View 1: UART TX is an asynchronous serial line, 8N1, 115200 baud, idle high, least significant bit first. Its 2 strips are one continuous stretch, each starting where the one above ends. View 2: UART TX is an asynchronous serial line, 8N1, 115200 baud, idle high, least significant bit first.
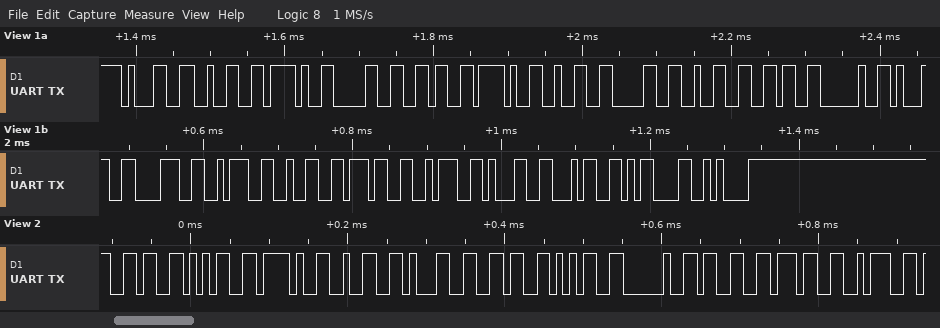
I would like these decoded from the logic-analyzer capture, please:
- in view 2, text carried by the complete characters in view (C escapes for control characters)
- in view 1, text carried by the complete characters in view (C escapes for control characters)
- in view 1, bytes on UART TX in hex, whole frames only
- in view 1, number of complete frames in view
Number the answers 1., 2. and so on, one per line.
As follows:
1. "65/2165 37:"
2. "12/06/2026 18:27:14\r\n"
3. 0x31 0x32 0x2F 0x30 0x36 0x2F 0x32 0x30 0x32 0x36 0x20 0x31 0x38 0x3A 0x32 0x37 0x3A 0x31 0x34 0x0D 0x0A
4. 21
